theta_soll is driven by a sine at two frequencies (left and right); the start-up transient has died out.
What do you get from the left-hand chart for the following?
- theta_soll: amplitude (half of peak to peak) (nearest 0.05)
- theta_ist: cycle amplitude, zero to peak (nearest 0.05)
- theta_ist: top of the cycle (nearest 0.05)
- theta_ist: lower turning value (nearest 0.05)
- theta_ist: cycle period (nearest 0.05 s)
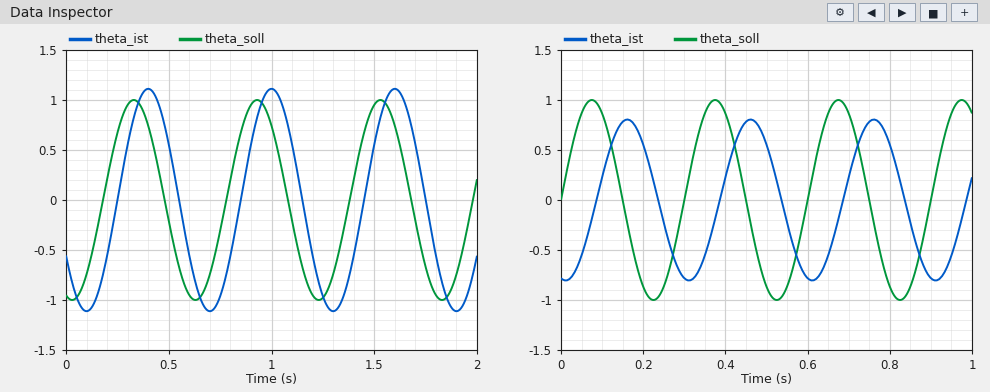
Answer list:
1.00
1.10
1.10
-1.10
0.60 s
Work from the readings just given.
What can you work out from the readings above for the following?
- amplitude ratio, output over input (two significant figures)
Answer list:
1.1
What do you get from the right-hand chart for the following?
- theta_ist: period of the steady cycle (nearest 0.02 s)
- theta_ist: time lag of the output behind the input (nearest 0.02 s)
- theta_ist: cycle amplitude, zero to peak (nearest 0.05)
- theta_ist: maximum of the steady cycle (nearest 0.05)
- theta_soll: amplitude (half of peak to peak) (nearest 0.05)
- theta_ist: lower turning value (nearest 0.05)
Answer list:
0.30 s
0.08 s
0.80
0.80
1.00
-0.80
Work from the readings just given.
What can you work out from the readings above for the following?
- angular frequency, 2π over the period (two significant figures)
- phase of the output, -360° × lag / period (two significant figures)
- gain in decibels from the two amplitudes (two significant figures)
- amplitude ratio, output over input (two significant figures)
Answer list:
21 rad/s
-96°
-1.9 dB
0.80
